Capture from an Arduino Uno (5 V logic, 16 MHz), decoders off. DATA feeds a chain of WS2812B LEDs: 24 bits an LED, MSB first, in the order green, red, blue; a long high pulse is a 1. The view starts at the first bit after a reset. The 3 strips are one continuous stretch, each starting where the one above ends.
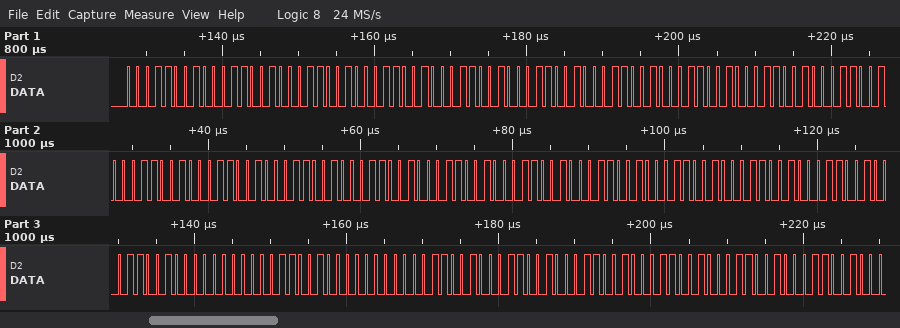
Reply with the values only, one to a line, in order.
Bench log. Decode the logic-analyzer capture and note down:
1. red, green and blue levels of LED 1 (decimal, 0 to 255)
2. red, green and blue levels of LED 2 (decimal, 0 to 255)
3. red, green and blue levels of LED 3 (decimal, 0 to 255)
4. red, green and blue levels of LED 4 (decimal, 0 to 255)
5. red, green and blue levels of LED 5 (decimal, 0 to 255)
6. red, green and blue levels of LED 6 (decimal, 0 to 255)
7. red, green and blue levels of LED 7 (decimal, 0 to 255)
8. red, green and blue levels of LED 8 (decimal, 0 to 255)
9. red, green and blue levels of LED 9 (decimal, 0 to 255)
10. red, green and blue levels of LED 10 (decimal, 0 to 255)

25, 25, 25
25, 25, 25
25, 25, 25
25, 25, 25
25, 25, 25
25, 25, 25
25, 25, 25
25, 0, 0
25, 25, 25
25, 25, 25
